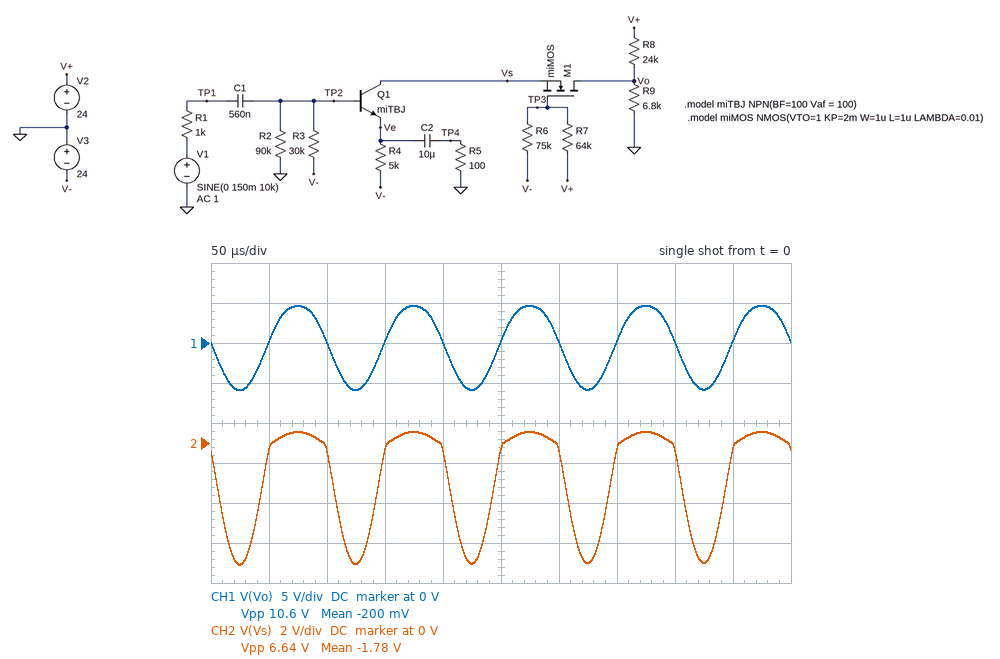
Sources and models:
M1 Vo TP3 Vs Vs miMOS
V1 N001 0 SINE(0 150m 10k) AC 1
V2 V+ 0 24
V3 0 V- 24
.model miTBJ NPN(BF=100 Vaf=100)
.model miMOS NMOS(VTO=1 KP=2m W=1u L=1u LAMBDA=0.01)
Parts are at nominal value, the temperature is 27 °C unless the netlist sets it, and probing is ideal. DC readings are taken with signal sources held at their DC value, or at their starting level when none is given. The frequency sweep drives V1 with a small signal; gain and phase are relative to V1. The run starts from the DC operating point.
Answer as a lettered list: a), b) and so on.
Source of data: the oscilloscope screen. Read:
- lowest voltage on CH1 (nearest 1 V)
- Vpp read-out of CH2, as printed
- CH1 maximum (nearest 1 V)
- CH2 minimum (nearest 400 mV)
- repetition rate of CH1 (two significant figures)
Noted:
a) -6 V
b) 6.64 V
c) 5 V
d) -6.0 V
e) 10 kHz
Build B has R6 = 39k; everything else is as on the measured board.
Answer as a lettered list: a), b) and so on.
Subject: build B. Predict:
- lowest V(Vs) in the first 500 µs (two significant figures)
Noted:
a) -8.3 V
